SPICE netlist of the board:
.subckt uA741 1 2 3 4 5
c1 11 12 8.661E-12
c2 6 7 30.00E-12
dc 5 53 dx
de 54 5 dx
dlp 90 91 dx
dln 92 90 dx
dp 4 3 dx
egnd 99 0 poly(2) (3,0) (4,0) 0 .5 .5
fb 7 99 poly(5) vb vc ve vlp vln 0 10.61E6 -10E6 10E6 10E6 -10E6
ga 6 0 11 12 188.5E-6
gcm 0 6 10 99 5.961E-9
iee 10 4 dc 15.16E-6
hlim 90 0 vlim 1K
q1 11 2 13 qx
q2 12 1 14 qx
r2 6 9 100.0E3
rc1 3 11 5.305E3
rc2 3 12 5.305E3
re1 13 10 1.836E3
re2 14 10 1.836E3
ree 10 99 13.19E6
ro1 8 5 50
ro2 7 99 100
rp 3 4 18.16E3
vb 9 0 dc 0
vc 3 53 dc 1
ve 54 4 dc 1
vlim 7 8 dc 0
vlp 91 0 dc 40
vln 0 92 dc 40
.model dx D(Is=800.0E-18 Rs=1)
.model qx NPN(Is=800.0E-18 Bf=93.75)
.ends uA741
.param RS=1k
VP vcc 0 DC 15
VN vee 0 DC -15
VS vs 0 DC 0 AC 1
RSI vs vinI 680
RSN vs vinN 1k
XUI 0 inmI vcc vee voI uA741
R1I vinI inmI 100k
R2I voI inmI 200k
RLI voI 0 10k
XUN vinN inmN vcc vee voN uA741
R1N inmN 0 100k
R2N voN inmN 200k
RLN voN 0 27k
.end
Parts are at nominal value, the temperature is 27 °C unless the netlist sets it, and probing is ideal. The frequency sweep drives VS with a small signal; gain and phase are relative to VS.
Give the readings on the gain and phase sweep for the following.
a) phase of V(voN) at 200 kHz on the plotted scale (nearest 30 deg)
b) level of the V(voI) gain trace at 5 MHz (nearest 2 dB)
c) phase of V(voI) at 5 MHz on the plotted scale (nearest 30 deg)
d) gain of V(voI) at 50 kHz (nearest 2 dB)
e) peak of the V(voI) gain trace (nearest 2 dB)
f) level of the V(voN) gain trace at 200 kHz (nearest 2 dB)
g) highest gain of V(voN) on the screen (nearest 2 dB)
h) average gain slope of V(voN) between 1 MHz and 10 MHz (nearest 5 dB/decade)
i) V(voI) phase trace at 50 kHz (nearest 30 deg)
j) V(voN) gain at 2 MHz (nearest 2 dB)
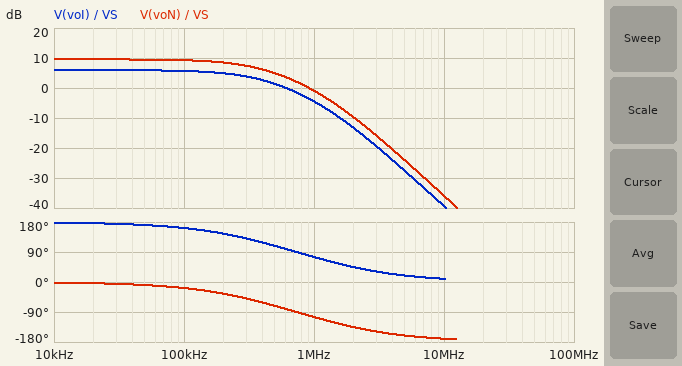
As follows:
-30 deg
-28 dB
30 deg
6 dB
6 dB
8 dB
10 dB
-35 dB/decade
180 deg
-10 dB
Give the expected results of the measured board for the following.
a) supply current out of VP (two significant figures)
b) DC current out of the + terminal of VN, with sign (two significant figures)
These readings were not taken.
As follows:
3.3 mA
-3.3 mA
